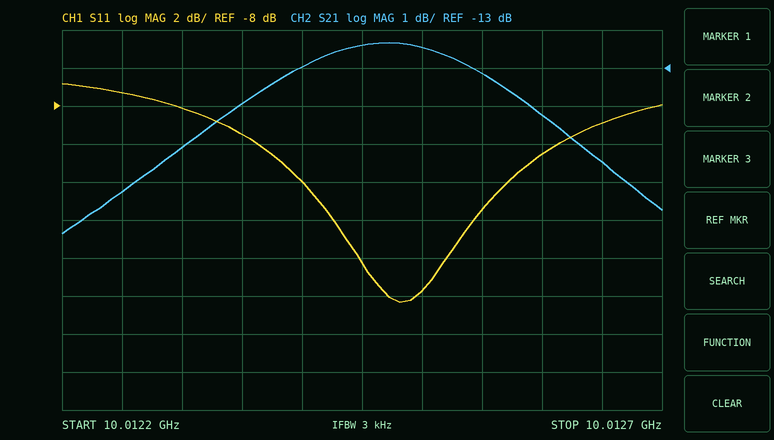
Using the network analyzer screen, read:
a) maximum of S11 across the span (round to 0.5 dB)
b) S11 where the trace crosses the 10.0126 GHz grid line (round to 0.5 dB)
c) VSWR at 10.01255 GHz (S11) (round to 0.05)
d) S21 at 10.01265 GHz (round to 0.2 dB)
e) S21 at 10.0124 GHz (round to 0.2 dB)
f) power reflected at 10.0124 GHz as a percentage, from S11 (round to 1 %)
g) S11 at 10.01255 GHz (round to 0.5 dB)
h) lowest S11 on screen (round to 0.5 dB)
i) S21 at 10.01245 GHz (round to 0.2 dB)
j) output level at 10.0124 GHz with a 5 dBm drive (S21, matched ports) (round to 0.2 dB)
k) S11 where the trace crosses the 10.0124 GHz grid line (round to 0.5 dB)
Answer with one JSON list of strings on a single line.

["-7.0 dB", "-10.5 dB", "1.55", "-15.4 dB", "-13.0 dB", "6 %", "-13.5 dB", "-18.5 dB", "-12.4 dB", "-8.0 dBm", "-12.0 dB"]
